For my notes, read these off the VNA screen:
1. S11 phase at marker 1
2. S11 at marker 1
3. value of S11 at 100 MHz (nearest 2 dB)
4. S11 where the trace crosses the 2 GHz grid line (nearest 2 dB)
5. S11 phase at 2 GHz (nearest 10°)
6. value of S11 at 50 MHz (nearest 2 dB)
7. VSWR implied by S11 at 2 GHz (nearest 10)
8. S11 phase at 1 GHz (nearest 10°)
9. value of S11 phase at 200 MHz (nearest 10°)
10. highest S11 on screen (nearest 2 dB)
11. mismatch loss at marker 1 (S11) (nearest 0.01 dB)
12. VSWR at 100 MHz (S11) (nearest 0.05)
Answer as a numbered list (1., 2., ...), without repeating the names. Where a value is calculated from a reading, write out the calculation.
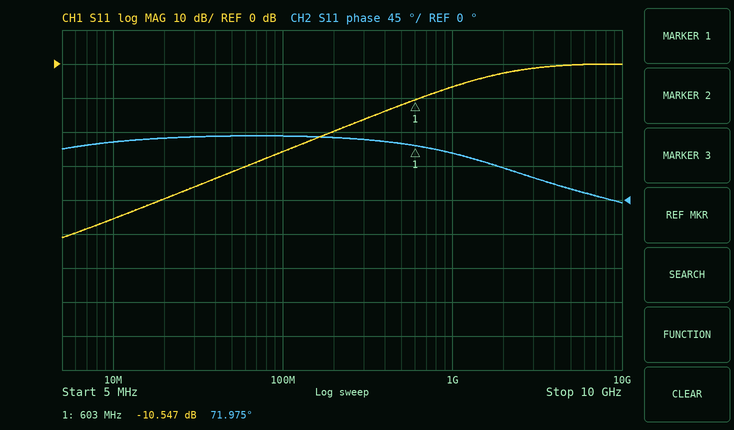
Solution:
1. 71.975°
2. -10.547 dB
3. -26 dB
4. -2 dB
5. 40°
6. -32 dB
7. |Γ| = 10^(-2/20) = 0.7943; VSWR = (1 + 0.7943)/(1 − 0.7943) ≈ 8.72, so 10 to the nearest 10
8. 60°
9. 80°
10. 0 dB
11. −10 log10(1 − 10^(-10.547/10)) ≈ 0.40 dB
12. |Γ| = 10^(-26/20) = 0.0501; VSWR = (1 + 0.0501)/(1 − 0.0501) ≈ 1.11, so 1.10 to the nearest 0.05
